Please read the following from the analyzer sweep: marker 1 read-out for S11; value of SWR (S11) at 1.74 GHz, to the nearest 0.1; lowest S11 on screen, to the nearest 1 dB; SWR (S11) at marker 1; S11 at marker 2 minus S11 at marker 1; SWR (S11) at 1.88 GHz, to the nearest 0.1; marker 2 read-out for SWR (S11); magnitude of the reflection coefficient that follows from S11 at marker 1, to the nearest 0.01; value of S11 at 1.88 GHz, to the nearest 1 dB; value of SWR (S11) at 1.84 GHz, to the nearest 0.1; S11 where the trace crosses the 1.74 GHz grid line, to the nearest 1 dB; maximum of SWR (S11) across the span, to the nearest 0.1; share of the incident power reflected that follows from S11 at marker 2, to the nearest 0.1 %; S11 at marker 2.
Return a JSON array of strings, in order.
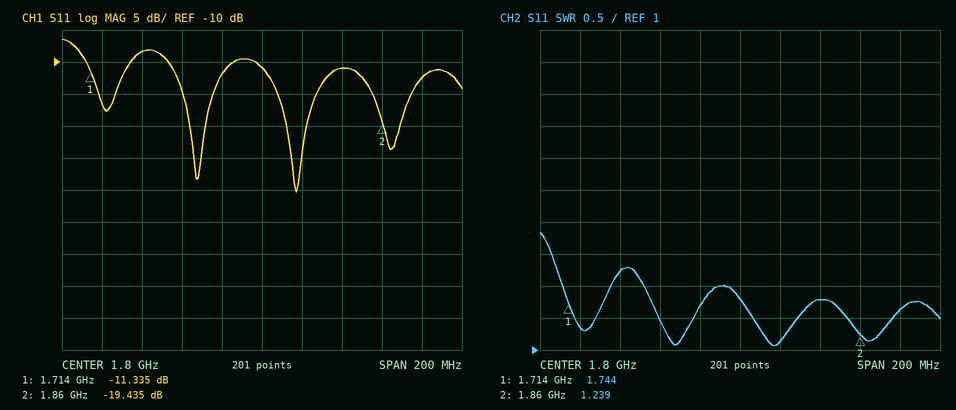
["-11.335 dB", "2.2", "-30 dB", "1.744", "-8.100 dB", "1.6", "1.239", "0.27", "-12 dB", "1.8", "-8 dB", "2.8", "1.1 %", "-19.435 dB"]
